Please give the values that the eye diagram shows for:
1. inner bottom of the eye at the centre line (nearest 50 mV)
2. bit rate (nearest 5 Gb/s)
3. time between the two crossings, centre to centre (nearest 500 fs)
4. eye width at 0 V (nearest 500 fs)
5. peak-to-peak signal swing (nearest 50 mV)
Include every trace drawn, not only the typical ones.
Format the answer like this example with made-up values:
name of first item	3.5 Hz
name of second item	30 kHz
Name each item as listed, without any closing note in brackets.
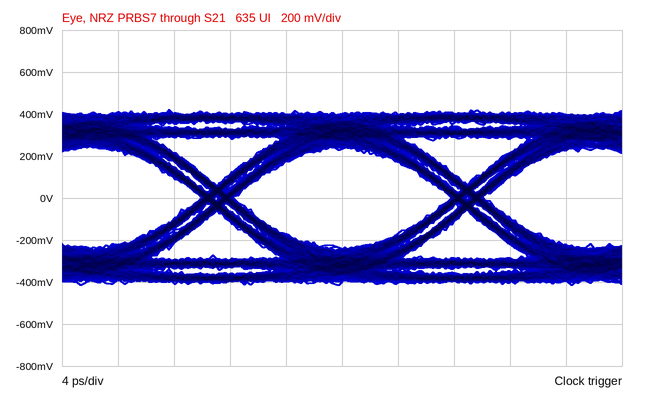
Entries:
inner bottom of the eye at the centre line	-250 mV
bit rate	55 Gb/s
time between the two crossings, centre to centre	18.0 ps
eye width at 0 V	15.5 ps
peak-to-peak signal swing	850 mV
